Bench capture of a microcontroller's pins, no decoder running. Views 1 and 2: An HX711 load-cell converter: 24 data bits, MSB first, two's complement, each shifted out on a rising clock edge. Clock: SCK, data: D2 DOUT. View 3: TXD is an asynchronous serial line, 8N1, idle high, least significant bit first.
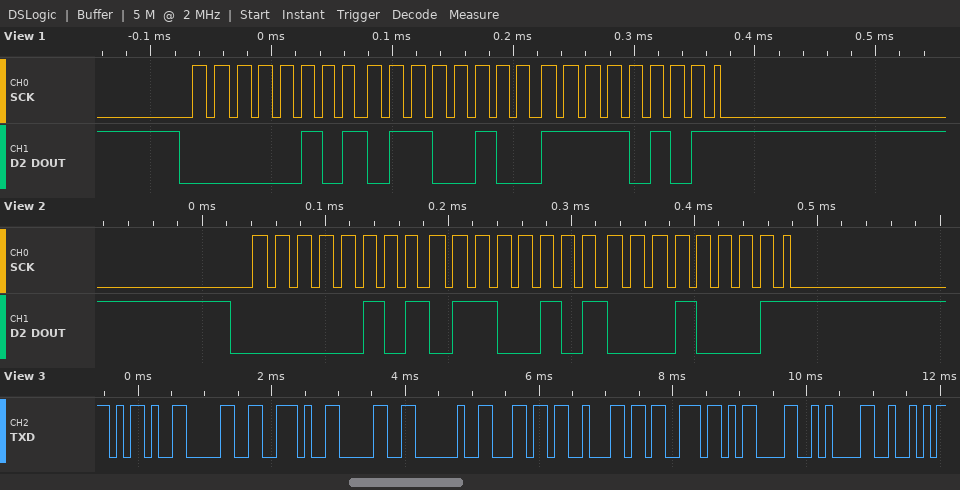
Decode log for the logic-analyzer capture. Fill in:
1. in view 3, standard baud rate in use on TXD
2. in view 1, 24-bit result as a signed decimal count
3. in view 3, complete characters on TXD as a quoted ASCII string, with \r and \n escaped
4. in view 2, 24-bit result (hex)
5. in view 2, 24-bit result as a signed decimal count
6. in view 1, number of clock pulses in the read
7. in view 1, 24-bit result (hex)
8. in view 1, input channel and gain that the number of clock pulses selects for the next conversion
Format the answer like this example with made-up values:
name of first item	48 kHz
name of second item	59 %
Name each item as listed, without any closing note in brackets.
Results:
in view 3, standard baud rate in use on TXD	9600 baud
in view 1, 24-bit result as a signed decimal count	353525
in view 3, complete characters on TXD as a quoted ASCII string, with \r and \n escaped	"-0.0 lbs\r\nR"
in view 2, 24-bit result	0x056511
in view 2, 24-bit result as a signed decimal count	353553
in view 1, number of clock pulses in the read	25
in view 1, 24-bit result	0x0564F5
in view 1, input channel and gain that the number of clock pulses selects for the next conversion	channel A, gain 128
